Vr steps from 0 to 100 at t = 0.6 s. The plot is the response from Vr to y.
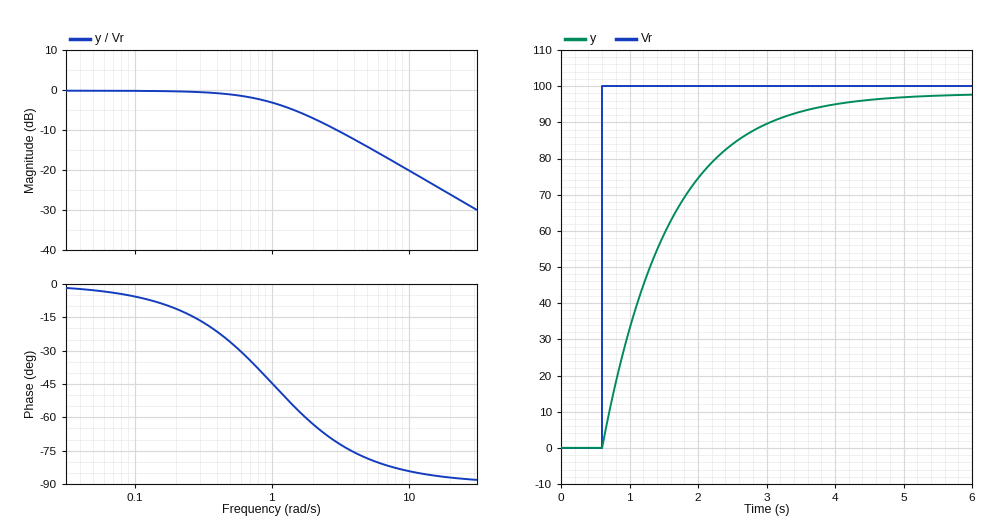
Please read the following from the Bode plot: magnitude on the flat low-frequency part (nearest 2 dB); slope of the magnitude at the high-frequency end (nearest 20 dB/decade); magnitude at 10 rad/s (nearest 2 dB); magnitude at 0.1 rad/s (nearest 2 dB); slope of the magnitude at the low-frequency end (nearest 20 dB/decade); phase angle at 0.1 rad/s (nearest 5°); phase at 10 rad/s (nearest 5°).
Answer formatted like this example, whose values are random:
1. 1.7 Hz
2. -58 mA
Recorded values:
1. 0 dB
2. -20 dB/decade
3. -20 dB
4. 0 dB
5. 0 dB/decade
6. -5°
7. -85°
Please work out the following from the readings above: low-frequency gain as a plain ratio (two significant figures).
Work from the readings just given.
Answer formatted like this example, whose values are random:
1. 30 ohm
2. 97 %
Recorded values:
1. 1.0
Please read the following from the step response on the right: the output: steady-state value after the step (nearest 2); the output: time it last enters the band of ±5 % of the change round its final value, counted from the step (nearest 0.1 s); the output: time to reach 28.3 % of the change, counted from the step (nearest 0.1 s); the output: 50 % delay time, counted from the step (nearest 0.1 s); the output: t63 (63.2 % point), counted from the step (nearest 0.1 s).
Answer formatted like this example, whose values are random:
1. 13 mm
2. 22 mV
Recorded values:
1. 98
2. 2.9 s
3. 0.3 s
4. 0.7 s
5. 1.0 s
